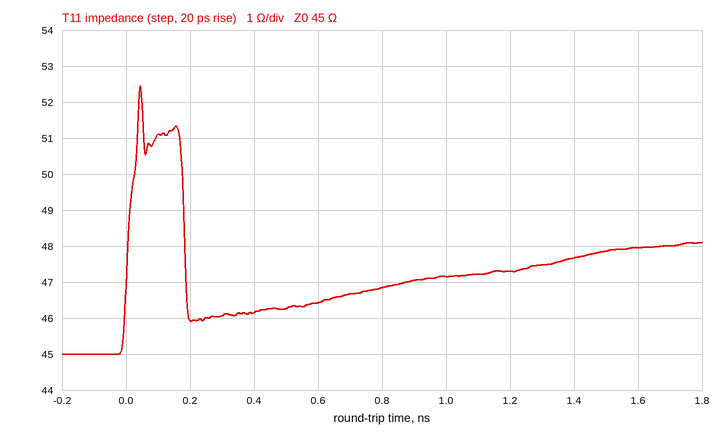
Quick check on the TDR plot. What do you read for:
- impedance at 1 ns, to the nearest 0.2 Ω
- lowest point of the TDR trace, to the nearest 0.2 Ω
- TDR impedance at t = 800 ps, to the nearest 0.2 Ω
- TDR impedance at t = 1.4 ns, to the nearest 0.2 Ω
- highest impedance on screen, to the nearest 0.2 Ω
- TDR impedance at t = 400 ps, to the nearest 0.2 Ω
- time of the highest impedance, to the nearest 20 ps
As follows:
47.2 Ω
45.0 Ω
46.8 Ω
47.6 Ω
52.4 Ω
46.2 Ω
40 ps
